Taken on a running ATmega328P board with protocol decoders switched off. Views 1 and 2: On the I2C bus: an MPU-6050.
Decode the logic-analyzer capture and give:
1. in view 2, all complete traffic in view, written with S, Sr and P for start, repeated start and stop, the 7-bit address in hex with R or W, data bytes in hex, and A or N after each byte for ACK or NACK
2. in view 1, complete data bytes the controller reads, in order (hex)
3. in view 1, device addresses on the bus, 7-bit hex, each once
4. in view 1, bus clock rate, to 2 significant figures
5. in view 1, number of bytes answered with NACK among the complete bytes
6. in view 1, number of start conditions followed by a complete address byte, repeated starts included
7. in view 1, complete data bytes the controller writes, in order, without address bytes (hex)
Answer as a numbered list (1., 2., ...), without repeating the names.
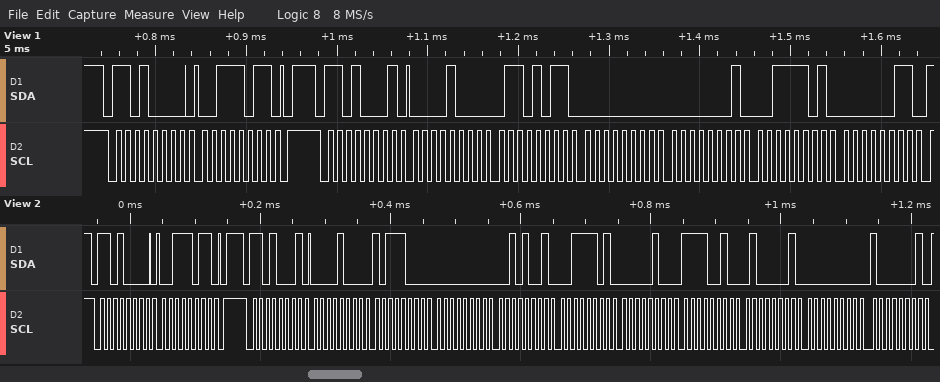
1. S 68W A 3B A P S 68R A 08 A B8 A 00 A 29 A 3D A 04 A F2 A 41 A 00 A 81 A
2. 08 6B 00 01 3D 03
3. 0x68
4. 100 kHz
5. 0
6. 2
7. 3B
